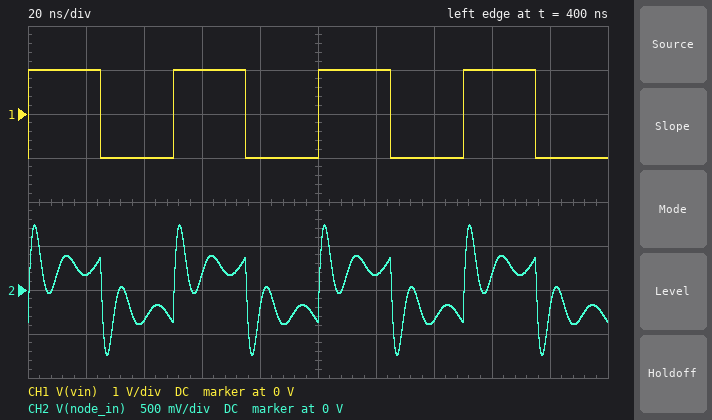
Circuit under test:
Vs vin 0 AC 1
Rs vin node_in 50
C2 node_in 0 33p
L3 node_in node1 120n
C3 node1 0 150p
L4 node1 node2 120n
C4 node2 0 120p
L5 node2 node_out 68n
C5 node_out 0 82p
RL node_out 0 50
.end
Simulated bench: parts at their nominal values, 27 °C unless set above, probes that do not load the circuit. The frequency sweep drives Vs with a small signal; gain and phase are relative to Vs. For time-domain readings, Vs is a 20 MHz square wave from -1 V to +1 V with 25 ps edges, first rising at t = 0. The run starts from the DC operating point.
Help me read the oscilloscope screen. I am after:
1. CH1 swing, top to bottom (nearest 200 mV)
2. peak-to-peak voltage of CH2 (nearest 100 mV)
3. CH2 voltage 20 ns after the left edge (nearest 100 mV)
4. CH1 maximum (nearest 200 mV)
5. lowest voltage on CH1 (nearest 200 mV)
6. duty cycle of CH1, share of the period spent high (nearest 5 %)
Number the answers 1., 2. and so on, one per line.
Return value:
1. 2.0 V
2. 1.5 V
3. 200 mV
4. 1.0 V
5. -1.0 V
6. 50 %
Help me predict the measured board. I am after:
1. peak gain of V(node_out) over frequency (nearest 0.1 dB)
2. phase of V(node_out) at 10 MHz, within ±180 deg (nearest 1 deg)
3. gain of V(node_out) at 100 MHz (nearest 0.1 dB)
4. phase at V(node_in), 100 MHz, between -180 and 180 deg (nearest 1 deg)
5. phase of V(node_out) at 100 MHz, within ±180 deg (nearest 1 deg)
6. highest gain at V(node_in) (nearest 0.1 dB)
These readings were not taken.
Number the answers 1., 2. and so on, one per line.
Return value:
1. -6.0 dB
2. -44 deg
3. -23.3 dB
4. -13 deg
5. -136 deg
6. -0.2 dB
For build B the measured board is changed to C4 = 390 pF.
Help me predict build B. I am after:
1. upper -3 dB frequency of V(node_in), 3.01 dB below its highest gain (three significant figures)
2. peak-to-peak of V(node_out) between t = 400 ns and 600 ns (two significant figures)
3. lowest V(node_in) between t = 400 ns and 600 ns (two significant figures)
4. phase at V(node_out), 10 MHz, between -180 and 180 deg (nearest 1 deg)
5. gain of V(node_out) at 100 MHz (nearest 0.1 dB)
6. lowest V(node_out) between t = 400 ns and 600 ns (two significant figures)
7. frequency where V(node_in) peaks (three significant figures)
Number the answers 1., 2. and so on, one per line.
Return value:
1. 144 MHz
2. 760 mV
3. -910 mV
4. -61 deg
5. -41.0 dB
6. -380 mV
7. 90.3 MHz
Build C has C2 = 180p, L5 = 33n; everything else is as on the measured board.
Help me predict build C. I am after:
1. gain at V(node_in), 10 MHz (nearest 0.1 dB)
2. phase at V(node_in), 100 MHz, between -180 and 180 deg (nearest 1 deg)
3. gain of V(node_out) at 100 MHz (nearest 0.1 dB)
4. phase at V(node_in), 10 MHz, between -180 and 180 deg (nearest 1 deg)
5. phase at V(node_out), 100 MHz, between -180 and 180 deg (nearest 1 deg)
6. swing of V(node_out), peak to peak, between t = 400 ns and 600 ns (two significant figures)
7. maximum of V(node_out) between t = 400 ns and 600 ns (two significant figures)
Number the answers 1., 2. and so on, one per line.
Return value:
1. -9.1 dB
2. -78 deg
3. -39.2 dB
4. -27 deg
5. -84 deg
6. 1.2 V
7. 600 mV
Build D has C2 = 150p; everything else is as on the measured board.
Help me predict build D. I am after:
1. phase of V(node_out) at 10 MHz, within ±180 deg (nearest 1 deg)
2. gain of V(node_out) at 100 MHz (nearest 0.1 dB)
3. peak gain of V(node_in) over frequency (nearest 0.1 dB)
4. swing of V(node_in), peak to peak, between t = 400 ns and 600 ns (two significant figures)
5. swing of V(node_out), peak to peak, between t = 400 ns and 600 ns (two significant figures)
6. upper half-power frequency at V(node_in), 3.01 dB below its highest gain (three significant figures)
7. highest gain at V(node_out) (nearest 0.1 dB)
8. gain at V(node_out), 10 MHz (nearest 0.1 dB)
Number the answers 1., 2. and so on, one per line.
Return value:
1. -51 deg
2. -35.1 dB
3. -4.4 dB
4. 850 mV
5. 1.3 V
6. 73.0 MHz
7. -6.0 dB
8. -7.0 dB
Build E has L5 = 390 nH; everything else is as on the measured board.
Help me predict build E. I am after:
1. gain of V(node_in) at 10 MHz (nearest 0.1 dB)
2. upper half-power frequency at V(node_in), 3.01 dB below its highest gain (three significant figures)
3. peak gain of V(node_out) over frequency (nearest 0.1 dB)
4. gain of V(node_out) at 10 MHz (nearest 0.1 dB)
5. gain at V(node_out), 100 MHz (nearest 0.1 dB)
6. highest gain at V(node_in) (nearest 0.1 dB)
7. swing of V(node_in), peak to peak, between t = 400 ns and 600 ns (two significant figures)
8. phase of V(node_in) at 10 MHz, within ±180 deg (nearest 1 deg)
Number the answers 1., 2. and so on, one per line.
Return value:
1. -6.7 dB
2. 144 MHz
3. -6.0 dB
4. -6.2 dB
5. -48.8 dB
6. 0 dB
7. 1.7 V
8. -10 deg
